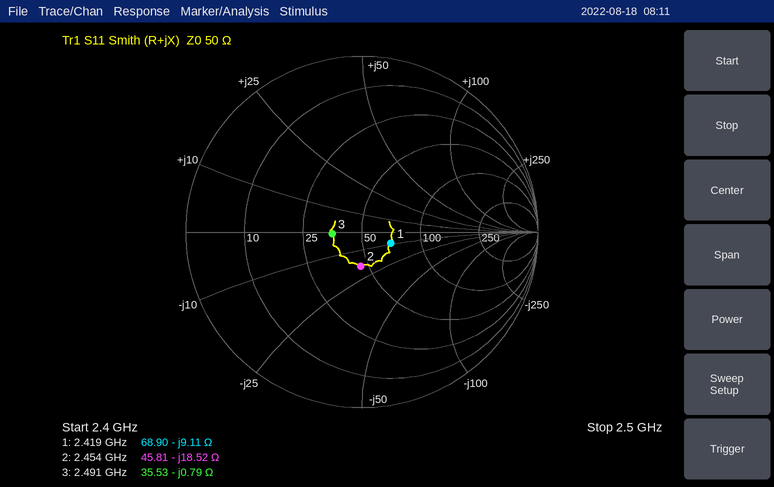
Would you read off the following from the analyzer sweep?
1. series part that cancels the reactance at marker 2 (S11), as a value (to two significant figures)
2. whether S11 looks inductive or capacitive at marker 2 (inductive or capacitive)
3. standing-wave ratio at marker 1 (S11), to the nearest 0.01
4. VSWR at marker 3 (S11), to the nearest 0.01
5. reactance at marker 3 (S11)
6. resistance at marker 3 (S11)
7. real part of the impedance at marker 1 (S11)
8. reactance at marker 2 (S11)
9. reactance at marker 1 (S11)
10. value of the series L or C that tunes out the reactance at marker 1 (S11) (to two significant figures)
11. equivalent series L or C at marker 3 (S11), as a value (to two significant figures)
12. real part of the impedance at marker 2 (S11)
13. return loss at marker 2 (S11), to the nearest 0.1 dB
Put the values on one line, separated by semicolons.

1.2 nH; capacitive; 1.43; 1.41; -0.79 Ω; 35.53 Ω; 68.90 Ω; -18.52 Ω; -9.11 Ω; 600 pH; 81 pF; 45.81 Ω; 14.2 dB
